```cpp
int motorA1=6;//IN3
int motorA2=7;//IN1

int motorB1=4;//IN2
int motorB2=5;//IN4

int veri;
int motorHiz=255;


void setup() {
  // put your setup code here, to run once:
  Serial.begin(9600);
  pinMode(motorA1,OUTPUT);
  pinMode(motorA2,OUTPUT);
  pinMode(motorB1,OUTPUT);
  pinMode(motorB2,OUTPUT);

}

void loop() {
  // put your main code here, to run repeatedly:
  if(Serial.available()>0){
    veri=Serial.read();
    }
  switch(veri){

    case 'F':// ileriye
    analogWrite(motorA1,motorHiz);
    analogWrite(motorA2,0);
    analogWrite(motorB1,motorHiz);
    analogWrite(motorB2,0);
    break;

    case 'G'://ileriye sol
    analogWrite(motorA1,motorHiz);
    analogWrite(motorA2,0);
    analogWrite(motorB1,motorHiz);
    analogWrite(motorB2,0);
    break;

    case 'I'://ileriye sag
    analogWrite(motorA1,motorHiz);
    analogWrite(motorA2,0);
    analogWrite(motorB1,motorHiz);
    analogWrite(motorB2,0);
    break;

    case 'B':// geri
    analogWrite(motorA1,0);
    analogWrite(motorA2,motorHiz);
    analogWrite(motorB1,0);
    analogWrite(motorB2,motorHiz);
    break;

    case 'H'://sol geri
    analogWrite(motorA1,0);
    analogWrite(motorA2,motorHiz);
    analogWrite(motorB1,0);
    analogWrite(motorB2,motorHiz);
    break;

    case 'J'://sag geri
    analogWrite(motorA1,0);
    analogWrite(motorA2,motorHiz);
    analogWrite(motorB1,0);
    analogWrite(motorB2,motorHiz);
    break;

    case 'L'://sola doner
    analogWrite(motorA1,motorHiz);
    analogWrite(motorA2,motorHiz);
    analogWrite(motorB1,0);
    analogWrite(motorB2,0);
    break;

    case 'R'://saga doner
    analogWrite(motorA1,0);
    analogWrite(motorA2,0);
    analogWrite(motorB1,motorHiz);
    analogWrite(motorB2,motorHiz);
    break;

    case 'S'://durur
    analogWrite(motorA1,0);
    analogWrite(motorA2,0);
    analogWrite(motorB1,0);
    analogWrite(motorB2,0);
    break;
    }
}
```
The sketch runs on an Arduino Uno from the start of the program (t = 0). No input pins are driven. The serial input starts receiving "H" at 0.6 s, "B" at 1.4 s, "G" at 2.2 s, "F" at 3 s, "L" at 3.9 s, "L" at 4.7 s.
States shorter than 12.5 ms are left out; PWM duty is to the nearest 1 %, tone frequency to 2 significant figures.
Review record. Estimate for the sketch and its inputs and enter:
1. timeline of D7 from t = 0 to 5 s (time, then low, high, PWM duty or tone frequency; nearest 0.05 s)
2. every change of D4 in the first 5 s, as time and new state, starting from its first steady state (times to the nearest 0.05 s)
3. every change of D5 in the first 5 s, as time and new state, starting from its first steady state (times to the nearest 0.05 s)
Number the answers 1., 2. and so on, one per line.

1. 0 s low; 0.6 s high; 2.2 s low; 3.9 s high
2. 0 s low; 2.2 s high; 3.9 s low
3. 0 s low; 0.6 s high; 2.2 s low
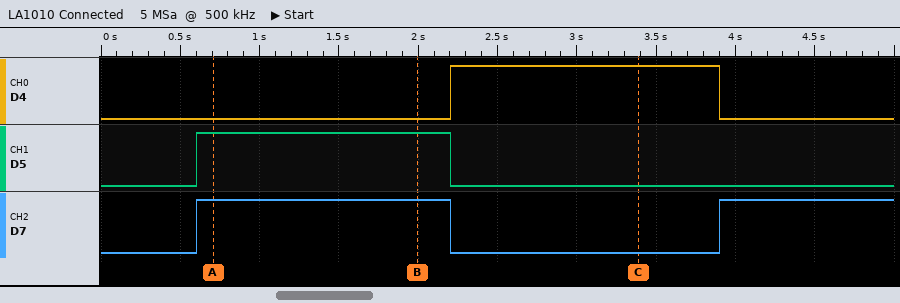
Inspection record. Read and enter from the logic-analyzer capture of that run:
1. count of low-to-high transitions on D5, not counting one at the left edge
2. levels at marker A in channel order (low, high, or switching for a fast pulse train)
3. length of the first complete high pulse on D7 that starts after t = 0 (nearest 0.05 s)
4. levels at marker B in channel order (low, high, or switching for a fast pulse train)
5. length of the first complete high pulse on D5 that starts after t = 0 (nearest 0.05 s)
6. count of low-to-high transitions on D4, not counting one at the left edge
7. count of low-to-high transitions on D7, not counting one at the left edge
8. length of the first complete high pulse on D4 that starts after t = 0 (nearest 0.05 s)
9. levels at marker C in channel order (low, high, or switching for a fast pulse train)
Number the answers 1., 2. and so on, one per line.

1. 1
2. D4 low, D5 high, D7 high
3. 1.60 s
4. D4 low, D5 high, D7 high
5. 1.60 s
6. 1
7. 2
8. 1.70 s
9. D4 high, D5 low, D7 low
